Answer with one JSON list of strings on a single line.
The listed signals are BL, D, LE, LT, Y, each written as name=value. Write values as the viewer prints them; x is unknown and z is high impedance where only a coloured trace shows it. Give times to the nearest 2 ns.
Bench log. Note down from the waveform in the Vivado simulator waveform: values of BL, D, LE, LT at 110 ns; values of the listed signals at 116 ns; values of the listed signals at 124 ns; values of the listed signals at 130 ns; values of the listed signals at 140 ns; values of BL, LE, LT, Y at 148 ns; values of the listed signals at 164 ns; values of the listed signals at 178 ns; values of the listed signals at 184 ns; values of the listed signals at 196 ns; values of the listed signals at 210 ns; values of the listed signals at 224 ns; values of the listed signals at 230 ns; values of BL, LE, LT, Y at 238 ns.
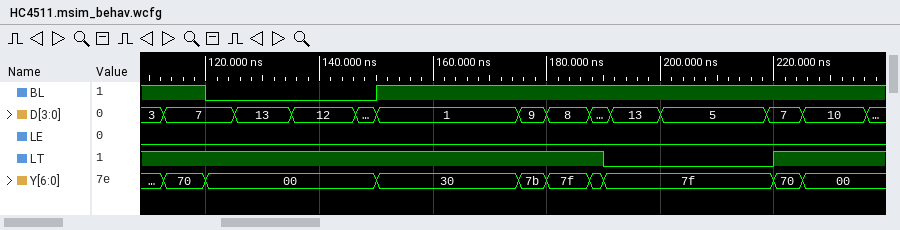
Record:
["BL=1, D=3, LE=0, LT=1", "BL=1, D=7, LE=0, LT=1, Y=70", "BL=0, D=7, LE=0, LT=1, Y=00", "BL=0, D=13, LE=0, LT=1, Y=00", "BL=0, D=12, LE=0, LT=1, Y=00", "BL=0, LE=0, LT=1, Y=00", "BL=1, D=1, LE=0, LT=1, Y=30", "BL=1, D=9, LE=0, LT=1, Y=7b", "BL=1, D=8, LE=0, LT=1, Y=7f", "BL=1, D=13, LE=0, LT=0, Y=7f", "BL=1, D=5, LE=0, LT=0, Y=7f", "BL=1, D=7, LE=0, LT=1, Y=70", "BL=1, D=10, LE=0, LT=1, Y=00", "BL=1, LE=0, LT=1, Y=00"]
